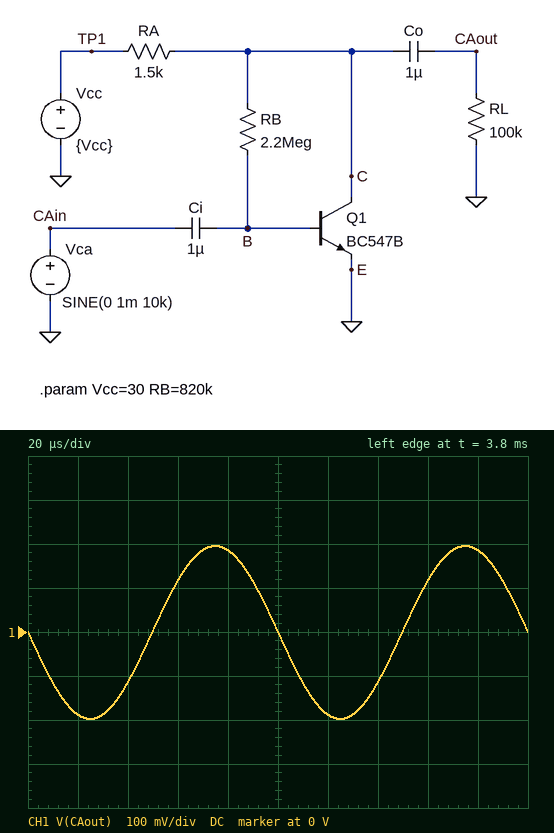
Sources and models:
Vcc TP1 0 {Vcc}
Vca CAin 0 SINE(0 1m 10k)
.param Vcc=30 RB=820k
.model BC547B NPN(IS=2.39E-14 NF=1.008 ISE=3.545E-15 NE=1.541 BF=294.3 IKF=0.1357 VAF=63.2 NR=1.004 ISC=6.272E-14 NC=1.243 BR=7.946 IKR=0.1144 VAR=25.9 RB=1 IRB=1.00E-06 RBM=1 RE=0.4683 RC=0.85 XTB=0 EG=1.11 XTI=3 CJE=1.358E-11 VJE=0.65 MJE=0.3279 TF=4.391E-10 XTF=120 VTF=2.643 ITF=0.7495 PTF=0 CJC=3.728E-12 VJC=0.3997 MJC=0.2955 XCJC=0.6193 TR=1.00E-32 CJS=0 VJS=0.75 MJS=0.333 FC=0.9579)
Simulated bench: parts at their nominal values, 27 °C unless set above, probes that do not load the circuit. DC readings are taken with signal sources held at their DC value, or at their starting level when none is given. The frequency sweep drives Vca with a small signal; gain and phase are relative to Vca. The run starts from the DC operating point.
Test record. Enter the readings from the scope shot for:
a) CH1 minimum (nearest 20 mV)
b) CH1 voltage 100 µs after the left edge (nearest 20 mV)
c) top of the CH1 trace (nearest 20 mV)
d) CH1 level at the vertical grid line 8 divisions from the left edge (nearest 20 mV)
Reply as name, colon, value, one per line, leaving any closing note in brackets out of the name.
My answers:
CH1 minimum: -200 mV
CH1 voltage 100 µs after the left edge: 0 V
top of the CH1 trace: 200 mV
CH1 level at the vertical grid line 8 divisions from the left edge: 120 mV
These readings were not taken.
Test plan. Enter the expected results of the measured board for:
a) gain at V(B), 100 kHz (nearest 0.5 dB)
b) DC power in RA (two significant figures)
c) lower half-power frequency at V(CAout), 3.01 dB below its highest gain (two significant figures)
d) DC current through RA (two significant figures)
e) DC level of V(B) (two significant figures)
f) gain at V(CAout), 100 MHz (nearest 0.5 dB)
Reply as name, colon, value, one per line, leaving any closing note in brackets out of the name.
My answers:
gain at V(B), 100 kHz: 0 dB
DC power in RA: 25 mW
lower half-power frequency at V(CAout), 3.01 dB below its highest gain: 75 Hz
DC current through RA: 4.1 mA
DC level of V(B): 670 mV
gain at V(CAout), 100 MHz: 42.5 dB
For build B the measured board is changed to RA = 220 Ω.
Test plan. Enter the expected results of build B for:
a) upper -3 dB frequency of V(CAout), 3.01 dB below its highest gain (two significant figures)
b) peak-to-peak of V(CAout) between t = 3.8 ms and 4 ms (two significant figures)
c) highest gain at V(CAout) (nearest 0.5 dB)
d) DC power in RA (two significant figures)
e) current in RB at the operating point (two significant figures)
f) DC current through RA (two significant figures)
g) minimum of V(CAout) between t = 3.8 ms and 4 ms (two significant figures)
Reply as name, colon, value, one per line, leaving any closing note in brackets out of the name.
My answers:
upper -3 dB frequency of V(CAout), 3.01 dB below its highest gain: 450 MHz
peak-to-peak of V(CAout) between t = 3.8 ms and 4 ms: 77 mV
highest gain at V(CAout): 31.5 dB
DC power in RA: 5.9 mW
current in RB at the operating point: 13 µA
DC current through RA: 5.2 mA
minimum of V(CAout) between t = 3.8 ms and 4 ms: -39 mV
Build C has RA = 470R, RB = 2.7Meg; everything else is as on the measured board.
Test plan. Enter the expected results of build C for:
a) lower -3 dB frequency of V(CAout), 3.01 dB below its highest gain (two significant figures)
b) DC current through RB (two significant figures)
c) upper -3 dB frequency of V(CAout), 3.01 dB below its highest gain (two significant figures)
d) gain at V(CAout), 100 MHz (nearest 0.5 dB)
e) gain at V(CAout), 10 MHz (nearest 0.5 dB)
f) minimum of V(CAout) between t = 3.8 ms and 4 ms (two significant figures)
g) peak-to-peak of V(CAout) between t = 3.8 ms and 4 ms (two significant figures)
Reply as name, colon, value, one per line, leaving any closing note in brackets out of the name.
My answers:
lower -3 dB frequency of V(CAout), 3.01 dB below its highest gain: 62 Hz
DC current through RB: 10 µA
upper -3 dB frequency of V(CAout), 3.01 dB below its highest gain: 270 MHz
gain at V(CAout), 100 MHz: 36.0 dB
gain at V(CAout), 10 MHz: 36.5 dB
minimum of V(CAout) between t = 3.8 ms and 4 ms: -66 mV
peak-to-peak of V(CAout) between t = 3.8 ms and 4 ms: 130 mV
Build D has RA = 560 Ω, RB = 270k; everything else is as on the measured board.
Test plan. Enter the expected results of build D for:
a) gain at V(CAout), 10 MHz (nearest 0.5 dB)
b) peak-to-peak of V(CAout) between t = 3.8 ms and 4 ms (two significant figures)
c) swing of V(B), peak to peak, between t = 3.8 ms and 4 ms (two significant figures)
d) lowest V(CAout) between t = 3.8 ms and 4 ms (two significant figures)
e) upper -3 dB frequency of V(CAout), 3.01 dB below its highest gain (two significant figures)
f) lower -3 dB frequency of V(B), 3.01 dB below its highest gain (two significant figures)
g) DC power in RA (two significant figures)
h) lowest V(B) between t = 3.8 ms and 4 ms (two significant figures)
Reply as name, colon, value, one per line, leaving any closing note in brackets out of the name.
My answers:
gain at V(CAout), 10 MHz: 48.5 dB
peak-to-peak of V(CAout) between t = 3.8 ms and 4 ms: 540 mV
swing of V(B), peak to peak, between t = 3.8 ms and 4 ms: 2.0 mV
lowest V(CAout) between t = 3.8 ms and 4 ms: -270 mV
upper -3 dB frequency of V(CAout), 3.01 dB below its highest gain: 160 MHz
lower -3 dB frequency of V(B), 3.01 dB below its highest gain: 460 Hz
DC power in RA: 250 mW
lowest V(B) between t = 3.8 ms and 4 ms: 720 mV
